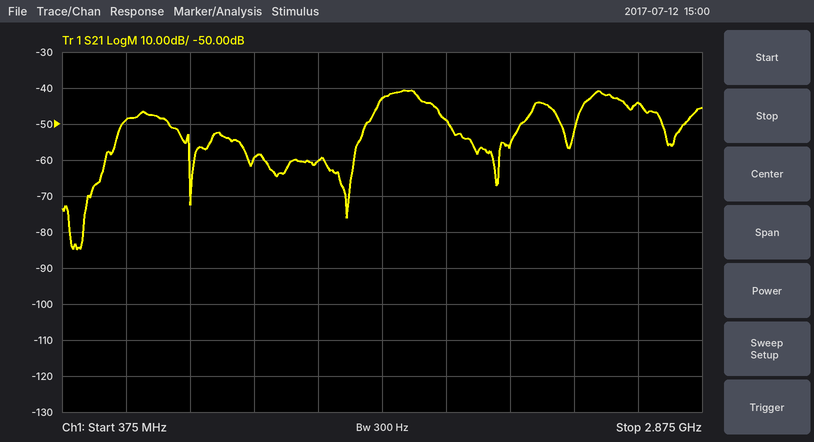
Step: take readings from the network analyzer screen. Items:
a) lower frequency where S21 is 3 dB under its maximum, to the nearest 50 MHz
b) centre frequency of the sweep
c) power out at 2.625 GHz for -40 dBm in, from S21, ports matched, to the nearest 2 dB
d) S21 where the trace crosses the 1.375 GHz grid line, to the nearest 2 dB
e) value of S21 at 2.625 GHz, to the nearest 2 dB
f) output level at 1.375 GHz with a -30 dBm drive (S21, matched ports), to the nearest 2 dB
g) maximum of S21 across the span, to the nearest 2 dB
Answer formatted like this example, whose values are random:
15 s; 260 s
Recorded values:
1.60 GHz; 1.625 GHz; -84 dBm; -60 dB; -44 dB; -90 dBm; -40 dB
